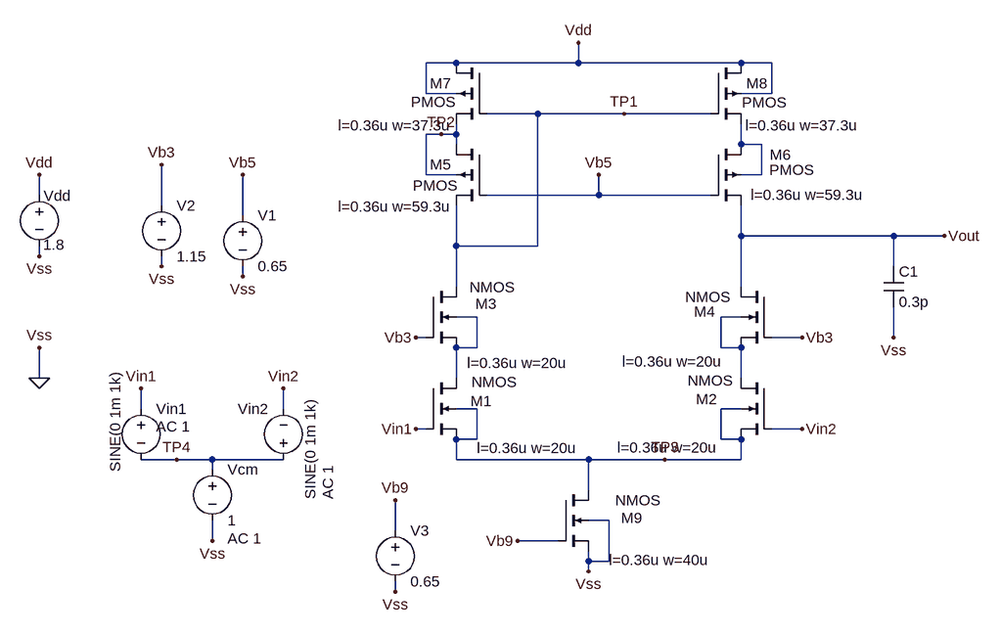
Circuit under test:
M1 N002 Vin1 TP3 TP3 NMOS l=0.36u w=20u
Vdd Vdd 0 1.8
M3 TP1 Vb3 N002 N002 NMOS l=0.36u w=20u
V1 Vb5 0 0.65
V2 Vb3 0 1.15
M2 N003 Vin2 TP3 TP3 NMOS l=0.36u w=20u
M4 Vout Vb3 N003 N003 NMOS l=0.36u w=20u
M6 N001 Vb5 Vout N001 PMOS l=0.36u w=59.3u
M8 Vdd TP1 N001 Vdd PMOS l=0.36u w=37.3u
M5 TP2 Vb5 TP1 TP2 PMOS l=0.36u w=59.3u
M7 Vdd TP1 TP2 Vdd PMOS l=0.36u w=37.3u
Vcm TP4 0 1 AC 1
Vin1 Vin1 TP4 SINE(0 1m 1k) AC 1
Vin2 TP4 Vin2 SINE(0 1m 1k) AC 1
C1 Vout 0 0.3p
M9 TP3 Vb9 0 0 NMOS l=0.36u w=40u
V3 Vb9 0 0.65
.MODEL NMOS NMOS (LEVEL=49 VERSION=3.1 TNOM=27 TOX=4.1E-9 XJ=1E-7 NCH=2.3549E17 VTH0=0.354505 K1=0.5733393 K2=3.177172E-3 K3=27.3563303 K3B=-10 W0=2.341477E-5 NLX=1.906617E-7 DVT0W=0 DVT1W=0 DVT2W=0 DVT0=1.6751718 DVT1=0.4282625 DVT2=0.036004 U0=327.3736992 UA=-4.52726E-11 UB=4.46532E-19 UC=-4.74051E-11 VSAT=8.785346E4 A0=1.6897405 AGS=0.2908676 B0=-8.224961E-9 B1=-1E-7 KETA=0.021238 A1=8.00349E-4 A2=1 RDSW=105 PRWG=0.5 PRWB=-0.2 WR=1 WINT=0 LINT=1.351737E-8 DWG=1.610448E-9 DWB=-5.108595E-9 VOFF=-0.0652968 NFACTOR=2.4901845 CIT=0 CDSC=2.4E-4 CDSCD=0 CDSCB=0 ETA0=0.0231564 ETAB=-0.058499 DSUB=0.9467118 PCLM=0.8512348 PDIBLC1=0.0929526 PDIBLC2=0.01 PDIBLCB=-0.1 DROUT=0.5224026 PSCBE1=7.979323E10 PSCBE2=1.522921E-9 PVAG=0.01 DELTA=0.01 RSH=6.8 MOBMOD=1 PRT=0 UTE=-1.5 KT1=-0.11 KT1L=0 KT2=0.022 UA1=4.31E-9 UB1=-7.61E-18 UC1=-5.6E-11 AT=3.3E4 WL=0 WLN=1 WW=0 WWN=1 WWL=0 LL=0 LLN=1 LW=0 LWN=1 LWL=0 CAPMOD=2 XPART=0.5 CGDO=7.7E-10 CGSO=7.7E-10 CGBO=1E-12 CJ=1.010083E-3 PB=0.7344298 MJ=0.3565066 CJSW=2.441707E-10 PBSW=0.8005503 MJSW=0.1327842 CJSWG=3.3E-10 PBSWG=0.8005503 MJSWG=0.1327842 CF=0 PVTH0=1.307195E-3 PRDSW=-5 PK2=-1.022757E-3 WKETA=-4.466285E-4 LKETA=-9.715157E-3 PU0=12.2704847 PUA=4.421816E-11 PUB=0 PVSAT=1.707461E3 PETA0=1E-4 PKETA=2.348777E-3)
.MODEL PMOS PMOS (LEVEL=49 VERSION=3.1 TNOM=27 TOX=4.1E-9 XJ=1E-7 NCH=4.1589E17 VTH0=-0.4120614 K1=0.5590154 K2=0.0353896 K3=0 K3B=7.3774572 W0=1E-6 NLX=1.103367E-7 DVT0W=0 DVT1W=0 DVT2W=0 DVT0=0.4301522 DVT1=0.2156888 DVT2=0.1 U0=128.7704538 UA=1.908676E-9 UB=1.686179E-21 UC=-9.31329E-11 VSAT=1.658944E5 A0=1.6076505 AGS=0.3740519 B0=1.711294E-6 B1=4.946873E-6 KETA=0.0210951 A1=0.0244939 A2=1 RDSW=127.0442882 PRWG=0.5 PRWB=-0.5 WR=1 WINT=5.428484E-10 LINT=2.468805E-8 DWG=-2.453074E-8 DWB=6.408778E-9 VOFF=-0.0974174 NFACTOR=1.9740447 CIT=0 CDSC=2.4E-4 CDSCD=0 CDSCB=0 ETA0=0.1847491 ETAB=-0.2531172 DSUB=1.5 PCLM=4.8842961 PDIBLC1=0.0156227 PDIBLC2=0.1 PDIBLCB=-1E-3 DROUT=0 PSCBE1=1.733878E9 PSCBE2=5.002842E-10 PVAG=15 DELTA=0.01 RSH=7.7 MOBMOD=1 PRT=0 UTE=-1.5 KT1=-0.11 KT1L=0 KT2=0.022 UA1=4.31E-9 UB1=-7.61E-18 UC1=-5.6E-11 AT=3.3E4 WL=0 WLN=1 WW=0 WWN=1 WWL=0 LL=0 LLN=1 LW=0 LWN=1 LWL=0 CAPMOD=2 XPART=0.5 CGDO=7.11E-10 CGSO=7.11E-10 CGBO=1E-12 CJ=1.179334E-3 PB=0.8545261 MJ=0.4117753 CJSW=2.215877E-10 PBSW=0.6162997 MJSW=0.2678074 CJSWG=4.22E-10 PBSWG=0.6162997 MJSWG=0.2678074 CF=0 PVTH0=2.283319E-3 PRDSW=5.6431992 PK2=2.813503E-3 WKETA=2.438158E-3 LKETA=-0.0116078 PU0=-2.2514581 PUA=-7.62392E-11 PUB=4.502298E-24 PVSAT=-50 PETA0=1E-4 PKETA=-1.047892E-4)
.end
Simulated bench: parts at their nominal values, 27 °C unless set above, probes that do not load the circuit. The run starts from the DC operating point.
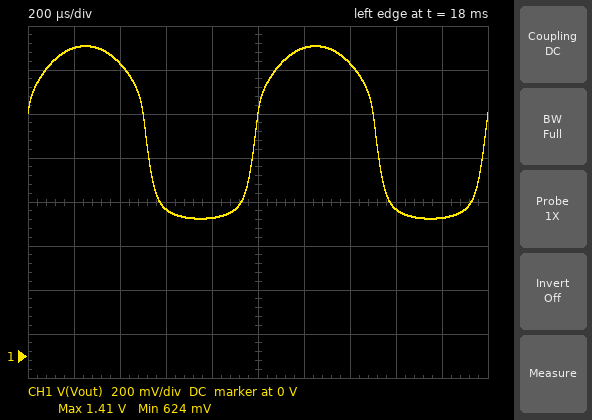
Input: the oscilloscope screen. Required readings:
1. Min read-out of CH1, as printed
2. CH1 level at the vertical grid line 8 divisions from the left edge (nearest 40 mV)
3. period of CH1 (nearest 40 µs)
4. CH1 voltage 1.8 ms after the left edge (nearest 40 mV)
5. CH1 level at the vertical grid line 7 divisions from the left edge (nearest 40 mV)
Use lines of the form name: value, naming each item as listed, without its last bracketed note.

Min read-out of CH1, as printed: 624 mV
CH1 level at the vertical grid line 8 divisions from the left edge: 680 mV
period of CH1: 1.00 ms
CH1 voltage 1.8 ms after the left edge: 640 mV
CH1 level at the vertical grid line 7 divisions from the left edge: 1.32 V
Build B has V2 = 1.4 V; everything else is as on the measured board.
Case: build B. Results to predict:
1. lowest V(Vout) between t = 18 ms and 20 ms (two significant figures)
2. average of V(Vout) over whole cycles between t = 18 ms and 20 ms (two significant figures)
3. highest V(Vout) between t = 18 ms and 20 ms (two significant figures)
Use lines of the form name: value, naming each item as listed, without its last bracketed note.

lowest V(Vout) between t = 18 ms and 20 ms: 680 mV
average of V(Vout) over whole cycles between t = 18 ms and 20 ms: 1.1 V
highest V(Vout) between t = 18 ms and 20 ms: 1.5 V
